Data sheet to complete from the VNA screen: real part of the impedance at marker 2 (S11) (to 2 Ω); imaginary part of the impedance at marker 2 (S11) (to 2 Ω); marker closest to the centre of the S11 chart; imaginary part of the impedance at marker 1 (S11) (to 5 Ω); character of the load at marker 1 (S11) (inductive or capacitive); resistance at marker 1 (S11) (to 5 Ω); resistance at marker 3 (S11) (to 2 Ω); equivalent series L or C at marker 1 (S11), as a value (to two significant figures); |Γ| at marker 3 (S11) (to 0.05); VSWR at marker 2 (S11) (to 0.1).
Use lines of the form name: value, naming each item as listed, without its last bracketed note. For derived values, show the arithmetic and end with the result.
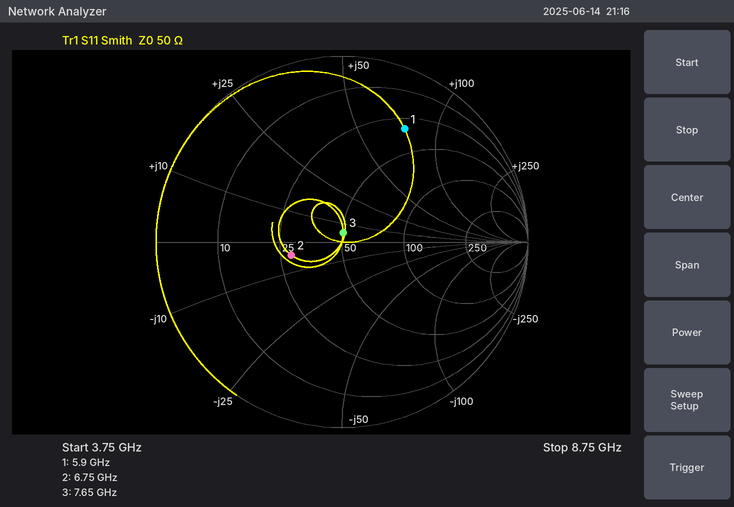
real part of the impedance at marker 2 (S11): 28 Ω
imaginary part of the impedance at marker 2 (S11): -4 Ω
marker closest to the centre of the S11 chart: marker 3
imaginary part of the impedance at marker 1 (S11): +75 Ω
character of the load at marker 1 (S11): inductive
resistance at marker 1 (S11): 30 Ω
resistance at marker 3 (S11): 50 Ω
equivalent series L or C at marker 1 (S11), as a value: L = 75 Ω/(2π × 5.9 GHz) ≈ 2.0 nH
|Γ| at marker 3 (S11): 0.05
VSWR at marker 2 (S11): 1.8
